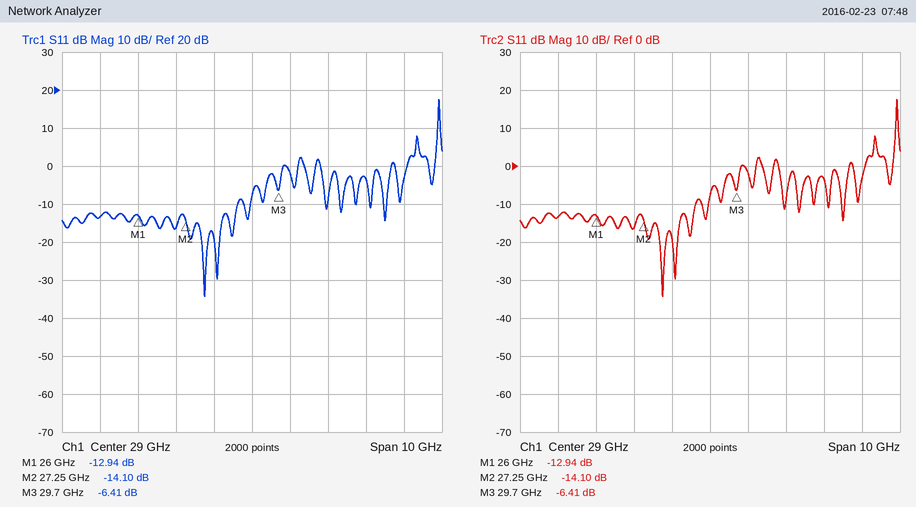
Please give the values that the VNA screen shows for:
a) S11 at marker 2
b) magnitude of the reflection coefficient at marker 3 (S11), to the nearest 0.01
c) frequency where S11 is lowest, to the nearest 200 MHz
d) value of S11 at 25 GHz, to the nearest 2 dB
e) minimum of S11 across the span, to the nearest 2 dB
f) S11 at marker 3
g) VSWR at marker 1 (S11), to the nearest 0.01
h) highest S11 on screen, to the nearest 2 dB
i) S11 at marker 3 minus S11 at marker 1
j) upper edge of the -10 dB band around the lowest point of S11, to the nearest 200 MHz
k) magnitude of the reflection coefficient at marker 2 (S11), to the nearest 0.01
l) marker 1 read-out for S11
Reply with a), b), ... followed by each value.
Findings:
a) -14.10 dB
b) 0.48
c) 27.8 GHz
d) -14 dB
e) -34 dB
f) -6.41 dB
g) 1.58
h) 18 dB
i) 6.53 dB
j) 28.6 GHz
k) 0.20
l) -12.94 dB
